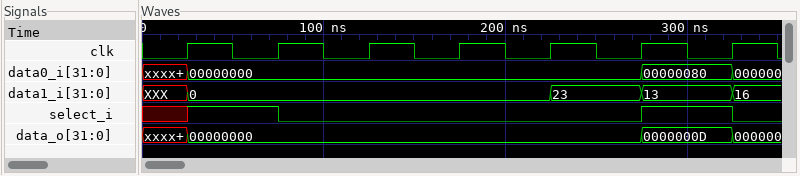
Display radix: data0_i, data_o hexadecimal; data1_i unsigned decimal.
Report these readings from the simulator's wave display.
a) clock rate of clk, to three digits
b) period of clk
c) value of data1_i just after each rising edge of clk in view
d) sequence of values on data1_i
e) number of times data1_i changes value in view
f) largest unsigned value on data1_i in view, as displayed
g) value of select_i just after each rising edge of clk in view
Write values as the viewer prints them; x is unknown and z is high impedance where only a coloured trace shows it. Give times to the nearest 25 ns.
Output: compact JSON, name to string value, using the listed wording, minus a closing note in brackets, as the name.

{"clock rate of clk, to three digits": "20.0 MHz", "period of clk": "50 ns", "value of data1_i just after each rising edge of clk in view": "0, 0, 0, 0, 23, 13, 16", "sequence of values on data1_i": "XXX, 0, 23, 13, 16", "number of times data1_i changes value in view": "4", "largest unsigned value on data1_i in view, as displayed": "23", "value of select_i just after each rising edge of clk in view": "1 0 0 0 0 1 0"}
